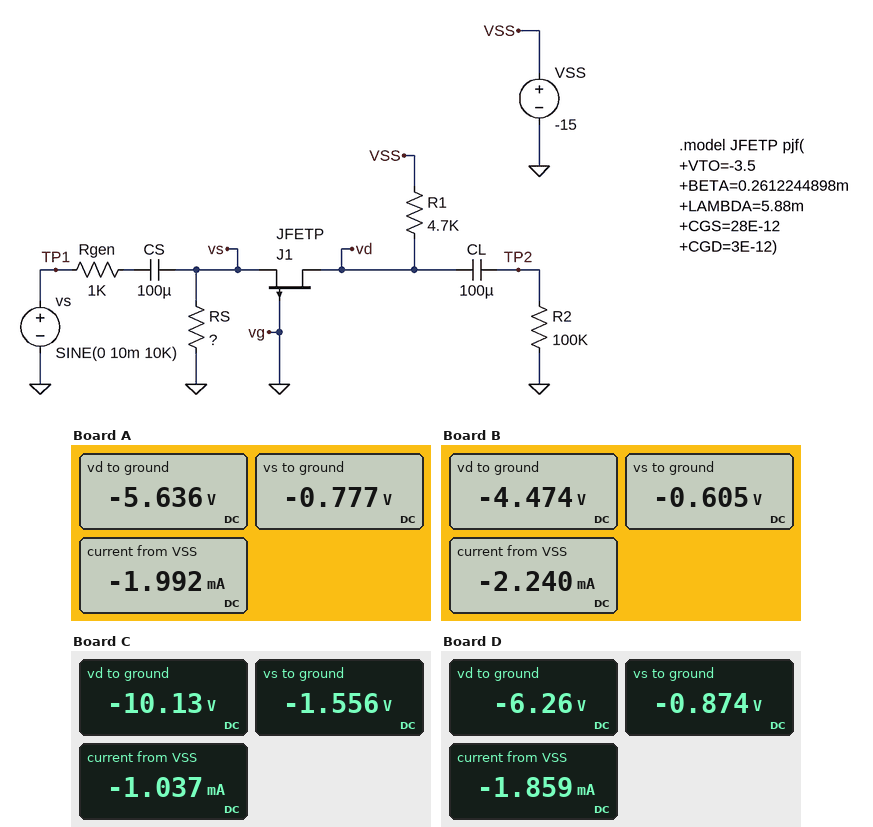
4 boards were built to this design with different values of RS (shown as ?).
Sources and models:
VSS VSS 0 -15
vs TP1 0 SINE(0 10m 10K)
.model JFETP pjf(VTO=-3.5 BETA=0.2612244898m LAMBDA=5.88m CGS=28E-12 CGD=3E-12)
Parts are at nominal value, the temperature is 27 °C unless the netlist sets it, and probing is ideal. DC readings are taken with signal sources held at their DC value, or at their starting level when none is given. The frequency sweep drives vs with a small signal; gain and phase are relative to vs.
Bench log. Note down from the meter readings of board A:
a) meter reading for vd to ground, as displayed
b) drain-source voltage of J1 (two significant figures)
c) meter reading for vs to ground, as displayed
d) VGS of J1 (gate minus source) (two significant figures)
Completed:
-5.636 V
-4.9 V
-0.777 V
780 mV
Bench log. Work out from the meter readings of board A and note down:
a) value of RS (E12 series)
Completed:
390 Ω
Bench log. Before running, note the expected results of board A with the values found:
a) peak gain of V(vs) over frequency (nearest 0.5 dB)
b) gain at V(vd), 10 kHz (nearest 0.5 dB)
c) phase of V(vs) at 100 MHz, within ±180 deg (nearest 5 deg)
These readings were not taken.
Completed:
-14.0 dB
2.0 dB
-70 deg
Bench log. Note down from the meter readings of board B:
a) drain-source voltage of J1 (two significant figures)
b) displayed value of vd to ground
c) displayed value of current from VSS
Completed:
-3.9 V
-4.474 V
-2.240 mA
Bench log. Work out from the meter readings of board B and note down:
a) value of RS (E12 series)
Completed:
270 Ω
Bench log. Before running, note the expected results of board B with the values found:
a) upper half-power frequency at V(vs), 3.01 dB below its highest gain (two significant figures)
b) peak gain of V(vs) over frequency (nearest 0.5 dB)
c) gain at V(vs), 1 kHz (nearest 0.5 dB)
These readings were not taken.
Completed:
44 MHz
-16.0 dB
-16.0 dB
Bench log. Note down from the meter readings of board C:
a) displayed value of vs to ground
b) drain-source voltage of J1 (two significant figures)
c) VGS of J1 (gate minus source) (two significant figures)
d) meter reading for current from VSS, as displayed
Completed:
-1.556 V
-8.6 V
1.6 V
-1.037 mA
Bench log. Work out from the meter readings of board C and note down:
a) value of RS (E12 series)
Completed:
1.5 kΩ
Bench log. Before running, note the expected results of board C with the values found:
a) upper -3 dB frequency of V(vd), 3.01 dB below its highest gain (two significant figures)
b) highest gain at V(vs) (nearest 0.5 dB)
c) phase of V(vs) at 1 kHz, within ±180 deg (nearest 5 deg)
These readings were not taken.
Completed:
19 MHz
-8.5 dB
0 deg
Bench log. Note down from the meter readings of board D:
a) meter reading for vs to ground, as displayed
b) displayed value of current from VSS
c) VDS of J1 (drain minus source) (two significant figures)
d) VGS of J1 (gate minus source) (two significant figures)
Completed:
-0.874 V
-1.859 mA
-5.4 V
870 mV
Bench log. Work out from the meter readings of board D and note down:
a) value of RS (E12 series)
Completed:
470 Ω
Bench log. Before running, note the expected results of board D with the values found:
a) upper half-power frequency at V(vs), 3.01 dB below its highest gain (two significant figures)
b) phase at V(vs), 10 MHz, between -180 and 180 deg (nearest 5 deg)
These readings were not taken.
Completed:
34 MHz
-15 deg
